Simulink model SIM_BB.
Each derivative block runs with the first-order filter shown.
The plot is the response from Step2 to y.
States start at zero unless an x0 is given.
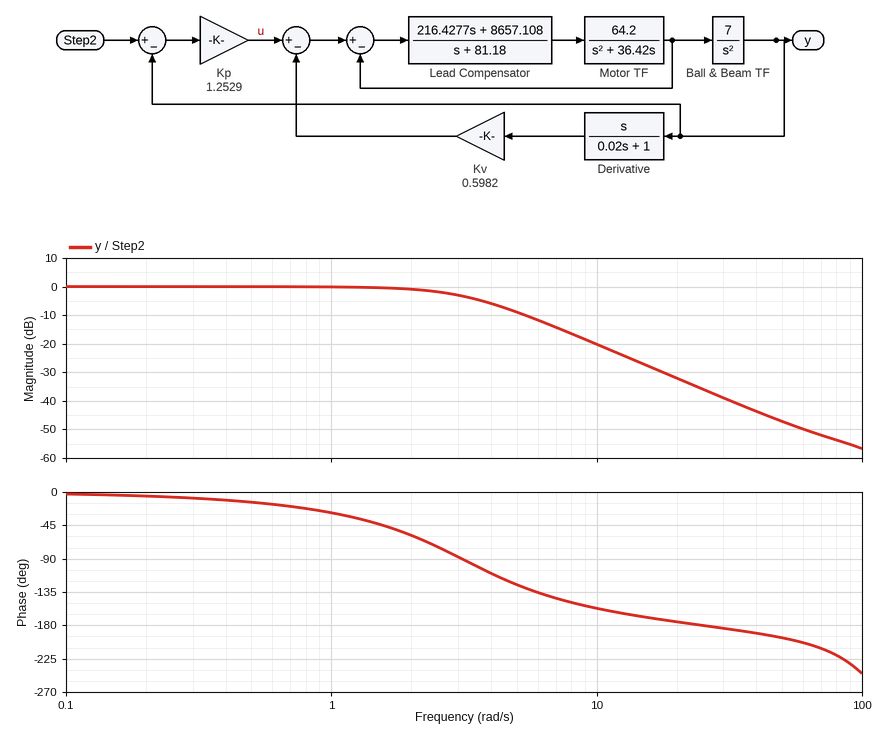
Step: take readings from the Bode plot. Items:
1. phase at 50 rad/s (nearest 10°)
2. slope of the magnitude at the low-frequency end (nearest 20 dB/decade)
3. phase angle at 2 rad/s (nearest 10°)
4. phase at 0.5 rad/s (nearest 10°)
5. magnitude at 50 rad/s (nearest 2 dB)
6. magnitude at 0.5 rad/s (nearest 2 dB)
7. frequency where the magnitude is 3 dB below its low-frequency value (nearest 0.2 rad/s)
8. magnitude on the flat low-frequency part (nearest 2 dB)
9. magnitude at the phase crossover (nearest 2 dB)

-200°
0 dB/decade
-60°
-10°
-48 dB
0 dB
3.0 rad/s
0 dB
-36 dB
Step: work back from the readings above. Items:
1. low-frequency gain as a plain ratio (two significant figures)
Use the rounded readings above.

1.0
